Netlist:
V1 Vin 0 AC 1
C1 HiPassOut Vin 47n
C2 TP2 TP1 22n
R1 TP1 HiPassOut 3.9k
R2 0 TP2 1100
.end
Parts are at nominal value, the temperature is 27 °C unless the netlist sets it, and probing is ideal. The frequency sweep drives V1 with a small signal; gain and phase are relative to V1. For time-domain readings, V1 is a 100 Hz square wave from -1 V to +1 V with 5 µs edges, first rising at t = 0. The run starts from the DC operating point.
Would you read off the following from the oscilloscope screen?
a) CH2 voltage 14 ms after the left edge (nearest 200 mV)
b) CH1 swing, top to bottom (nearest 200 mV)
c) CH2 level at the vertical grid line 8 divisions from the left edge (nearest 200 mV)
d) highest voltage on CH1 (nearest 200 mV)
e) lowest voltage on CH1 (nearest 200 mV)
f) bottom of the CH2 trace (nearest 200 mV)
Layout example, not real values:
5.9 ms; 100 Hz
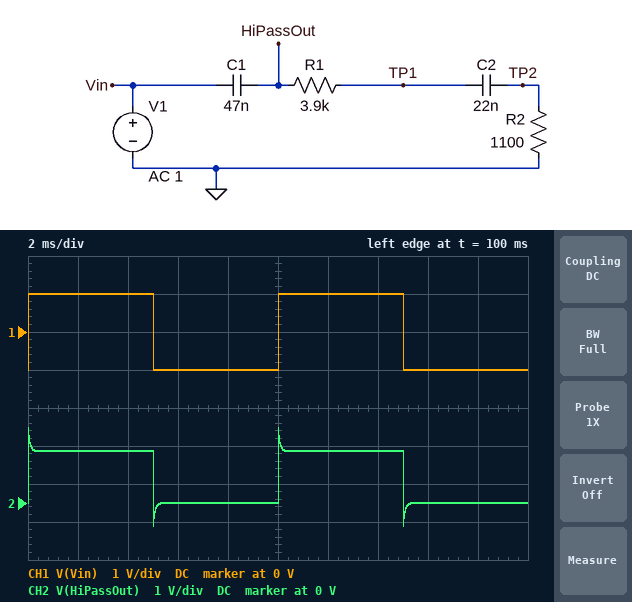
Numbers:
1.4 V; 2.0 V; 0 V; 1.0 V; -1.0 V; -600 mV
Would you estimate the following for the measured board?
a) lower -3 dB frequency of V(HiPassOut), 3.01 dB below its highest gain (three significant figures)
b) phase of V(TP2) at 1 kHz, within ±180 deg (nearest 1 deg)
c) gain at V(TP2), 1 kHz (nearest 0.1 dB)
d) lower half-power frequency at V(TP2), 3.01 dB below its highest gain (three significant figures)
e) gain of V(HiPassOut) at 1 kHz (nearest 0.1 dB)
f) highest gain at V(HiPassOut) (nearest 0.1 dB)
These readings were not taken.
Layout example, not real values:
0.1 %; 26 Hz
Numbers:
570 Hz; 65 deg; -20.6 dB; 2.12 kHz; -2.5 dB; 0 dB
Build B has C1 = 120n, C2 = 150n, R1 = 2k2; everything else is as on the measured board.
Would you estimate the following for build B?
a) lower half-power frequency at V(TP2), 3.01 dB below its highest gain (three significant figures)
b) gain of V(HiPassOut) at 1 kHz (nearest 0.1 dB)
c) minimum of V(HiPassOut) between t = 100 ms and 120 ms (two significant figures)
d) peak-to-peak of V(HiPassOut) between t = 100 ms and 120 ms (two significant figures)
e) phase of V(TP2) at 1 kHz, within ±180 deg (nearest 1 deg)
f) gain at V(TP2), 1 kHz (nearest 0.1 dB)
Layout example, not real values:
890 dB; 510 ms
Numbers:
723 Hz; -1.4 dB; -1.1 V; 3.1 V; 36 deg; -11.4 dB
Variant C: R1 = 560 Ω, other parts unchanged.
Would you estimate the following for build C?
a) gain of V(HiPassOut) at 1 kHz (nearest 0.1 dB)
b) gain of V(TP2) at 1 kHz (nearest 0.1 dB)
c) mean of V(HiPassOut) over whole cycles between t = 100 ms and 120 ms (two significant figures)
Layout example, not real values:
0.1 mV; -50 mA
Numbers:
-3.2 dB; -19.8 dB; 680 mV
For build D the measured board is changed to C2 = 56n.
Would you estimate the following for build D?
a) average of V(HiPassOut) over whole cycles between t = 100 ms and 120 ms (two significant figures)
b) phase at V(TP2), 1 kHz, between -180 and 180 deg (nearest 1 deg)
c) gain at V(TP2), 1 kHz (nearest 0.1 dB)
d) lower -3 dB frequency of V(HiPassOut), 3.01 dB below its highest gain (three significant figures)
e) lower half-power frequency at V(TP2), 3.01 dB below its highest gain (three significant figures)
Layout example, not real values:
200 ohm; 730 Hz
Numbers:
460 mV; 51 deg; -17.2 dB; 952 Hz; 1.25 kHz
